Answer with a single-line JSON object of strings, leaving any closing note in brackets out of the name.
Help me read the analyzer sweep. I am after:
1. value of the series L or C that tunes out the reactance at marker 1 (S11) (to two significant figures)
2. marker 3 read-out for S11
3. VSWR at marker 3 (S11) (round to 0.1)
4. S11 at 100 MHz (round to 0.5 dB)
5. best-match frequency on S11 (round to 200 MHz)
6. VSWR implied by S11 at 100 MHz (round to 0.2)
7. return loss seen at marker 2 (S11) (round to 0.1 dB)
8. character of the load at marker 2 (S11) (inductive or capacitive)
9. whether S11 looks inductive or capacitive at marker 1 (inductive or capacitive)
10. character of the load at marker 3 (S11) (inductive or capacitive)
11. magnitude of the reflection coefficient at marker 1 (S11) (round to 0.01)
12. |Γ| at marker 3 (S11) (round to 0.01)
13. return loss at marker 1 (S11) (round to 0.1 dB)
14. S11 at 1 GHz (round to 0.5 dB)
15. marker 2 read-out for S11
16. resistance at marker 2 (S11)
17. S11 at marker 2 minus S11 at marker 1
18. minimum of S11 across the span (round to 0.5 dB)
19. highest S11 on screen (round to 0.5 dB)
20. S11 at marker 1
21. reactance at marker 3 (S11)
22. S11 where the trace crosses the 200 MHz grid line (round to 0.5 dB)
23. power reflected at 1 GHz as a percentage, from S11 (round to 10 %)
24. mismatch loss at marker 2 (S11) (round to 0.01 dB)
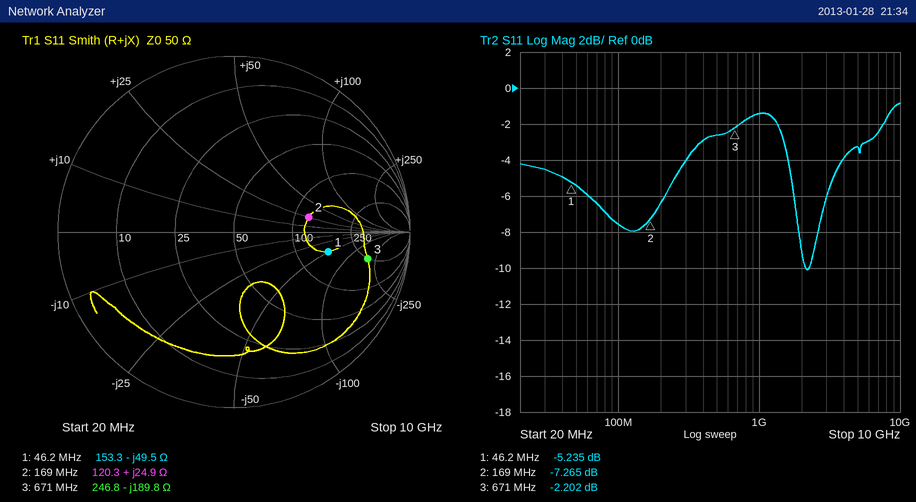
{"value of the series L or C that tunes out the reactance at marker 1 (S11)": "170 nH", "marker 3 read-out for S11": "-2.202 dB", "VSWR at marker 3 (S11)": "7.9", "S11 at 100 MHz": "-7.5 dB", "best-match frequency on S11": "2.2 GHz", "VSWR implied by S11 at 100 MHz": "2.4", "return loss seen at marker 2 (S11)": "7.3 dB", "character of the load at marker 2 (S11)": "inductive", "whether S11 looks inductive or capacitive at marker 1": "capacitive", "character of the load at marker 3 (S11)": "capacitive", "magnitude of the reflection coefficient at marker 1 (S11)": "0.55", "|Γ| at marker 3 (S11)": "0.78", "return loss at marker 1 (S11)": "5.2 dB", "S11 at 1 GHz": "-1.5 dB", "marker 2 read-out for S11": "-7.265 dB", "resistance at marker 2": "120.3 Ω", "S11 at marker 2 minus S11 at marker 1": "-2.030 dB", "minimum of S11 across the span": "-10.0 dB", "highest S11 on screen": "-1.0 dB", "S11 at marker 1": "-5.235 dB", "reactance at marker 3": "-189.8 Ω", "S11 where the trace crosses the 200 MHz grid line": "-6.5 dB", "power reflected at 1 GHz as a percentage, from S11": "70 %", "mismatch loss at marker 2 (S11)": "0.90 dB"}
